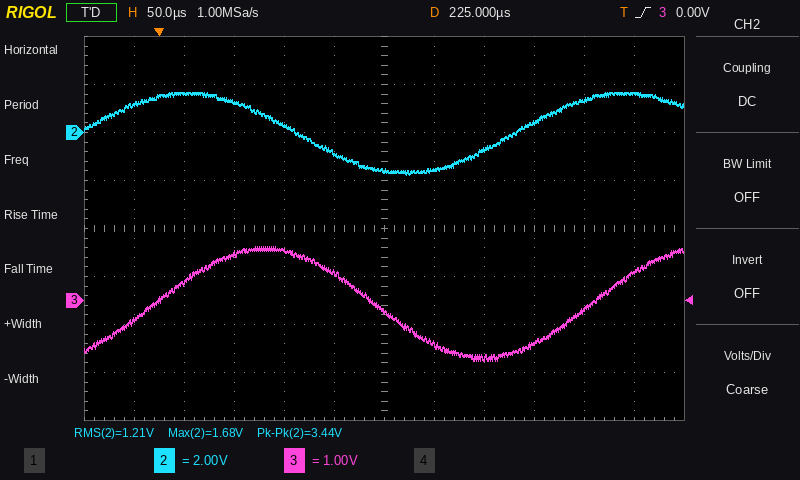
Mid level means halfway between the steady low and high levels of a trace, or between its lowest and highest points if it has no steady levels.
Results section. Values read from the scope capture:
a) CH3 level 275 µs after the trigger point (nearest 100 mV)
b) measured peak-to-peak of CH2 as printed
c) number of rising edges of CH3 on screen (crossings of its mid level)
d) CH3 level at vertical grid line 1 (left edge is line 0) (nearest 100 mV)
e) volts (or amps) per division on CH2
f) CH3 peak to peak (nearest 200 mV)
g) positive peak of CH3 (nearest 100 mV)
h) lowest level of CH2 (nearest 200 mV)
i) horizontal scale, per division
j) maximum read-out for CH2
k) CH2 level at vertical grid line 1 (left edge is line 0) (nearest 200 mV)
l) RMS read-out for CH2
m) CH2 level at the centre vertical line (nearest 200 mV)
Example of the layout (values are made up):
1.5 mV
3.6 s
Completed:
-900 mV
3.44 V
2
-400 mV
2 V
2.4 V
1.1 V
-1.8 V
50 µs
1.68 V
1.2 V
1.21 V
-1.6 V
